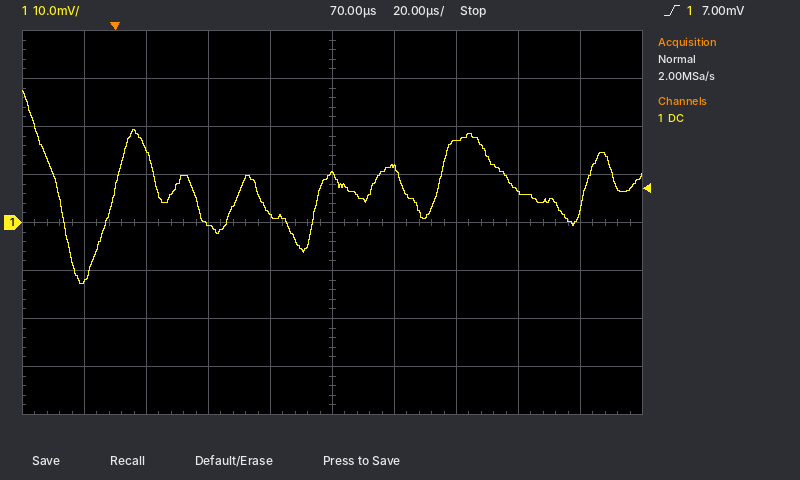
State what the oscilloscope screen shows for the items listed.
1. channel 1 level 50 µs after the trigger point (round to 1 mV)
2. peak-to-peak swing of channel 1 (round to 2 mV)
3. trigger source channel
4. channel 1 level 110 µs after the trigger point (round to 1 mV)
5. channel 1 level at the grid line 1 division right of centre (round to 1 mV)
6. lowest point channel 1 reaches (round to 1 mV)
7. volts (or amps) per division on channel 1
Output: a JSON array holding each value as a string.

["2 mV", "40 mV", "channel 1", "17 mV", "11 mV", "-13 mV", "10 mV"]
